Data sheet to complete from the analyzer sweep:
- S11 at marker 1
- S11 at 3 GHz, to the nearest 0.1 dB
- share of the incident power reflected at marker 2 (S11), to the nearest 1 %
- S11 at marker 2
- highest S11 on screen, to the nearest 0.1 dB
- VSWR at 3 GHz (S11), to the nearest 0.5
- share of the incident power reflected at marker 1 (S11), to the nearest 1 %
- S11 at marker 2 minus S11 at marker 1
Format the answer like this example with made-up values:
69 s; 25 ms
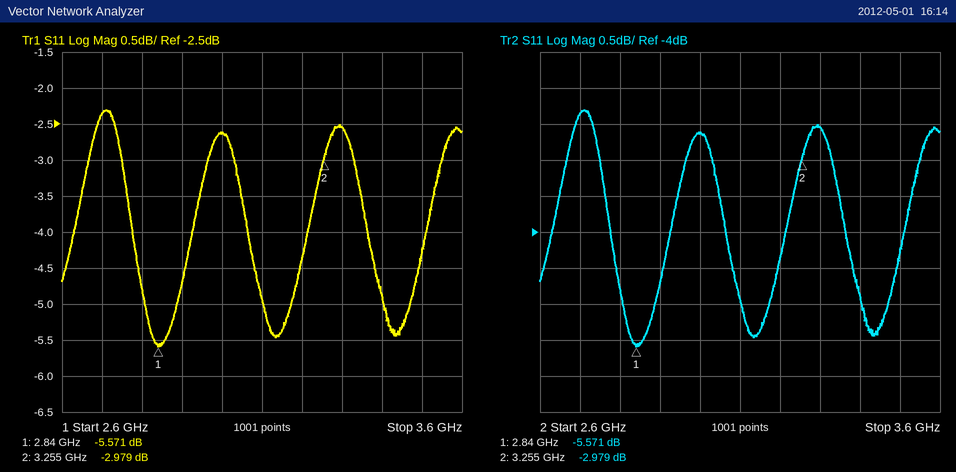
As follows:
-5.571 dB; -2.6 dB; 50 %; -2.979 dB; -2.3 dB; 6.5; 28 %; 2.592 dB
